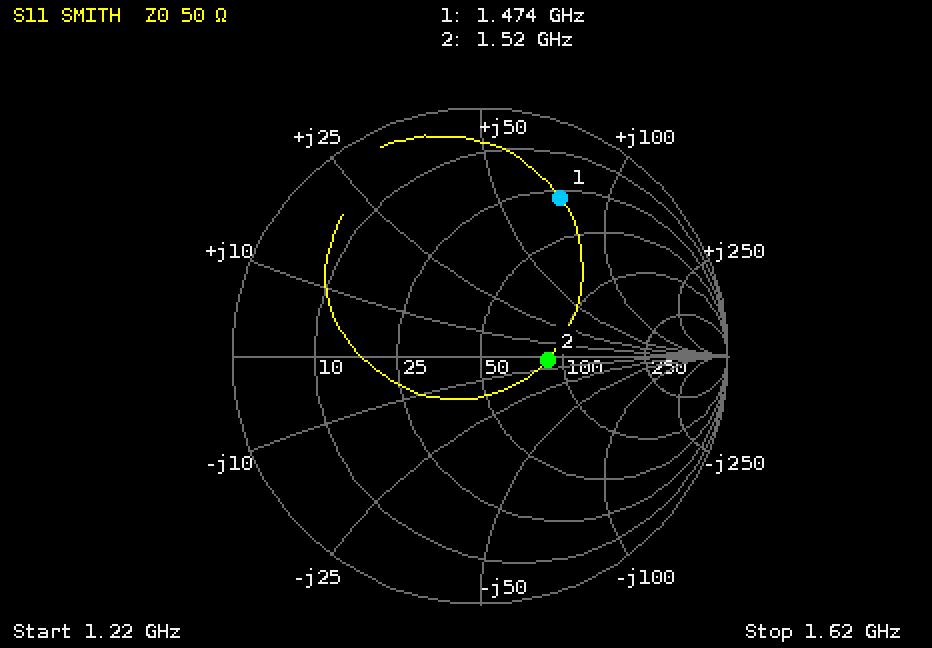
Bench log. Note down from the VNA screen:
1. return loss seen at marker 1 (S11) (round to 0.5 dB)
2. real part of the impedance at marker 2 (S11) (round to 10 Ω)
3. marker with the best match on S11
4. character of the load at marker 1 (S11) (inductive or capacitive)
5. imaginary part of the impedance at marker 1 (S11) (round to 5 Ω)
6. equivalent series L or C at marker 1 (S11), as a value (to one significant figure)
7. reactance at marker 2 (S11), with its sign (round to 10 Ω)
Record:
3.0 dB
90 Ω
marker 2
inductive
+75 Ω
8 nH
0 Ω
